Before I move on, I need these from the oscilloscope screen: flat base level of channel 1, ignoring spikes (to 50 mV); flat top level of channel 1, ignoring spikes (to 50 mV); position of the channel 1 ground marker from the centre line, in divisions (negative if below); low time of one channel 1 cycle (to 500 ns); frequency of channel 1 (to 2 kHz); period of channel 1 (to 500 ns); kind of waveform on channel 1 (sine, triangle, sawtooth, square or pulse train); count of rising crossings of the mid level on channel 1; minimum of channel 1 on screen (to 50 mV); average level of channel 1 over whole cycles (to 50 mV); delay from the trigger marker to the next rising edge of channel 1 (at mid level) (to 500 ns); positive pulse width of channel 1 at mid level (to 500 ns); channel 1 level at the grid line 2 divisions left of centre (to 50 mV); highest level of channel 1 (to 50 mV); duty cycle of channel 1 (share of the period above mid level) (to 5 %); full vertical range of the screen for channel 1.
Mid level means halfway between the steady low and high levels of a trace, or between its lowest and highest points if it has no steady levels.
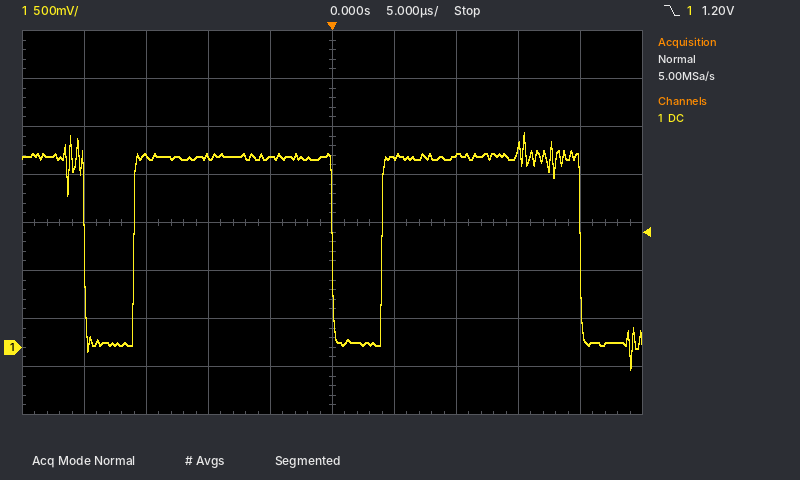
50 mV
2.00 V
-2.6 div
4.0 µs
50 kHz
20.0 µs
pulse train
2
-250 mV
1.60 V
4.0 µs
16.0 µs
2.00 V
2.25 V
80 %
4 V
